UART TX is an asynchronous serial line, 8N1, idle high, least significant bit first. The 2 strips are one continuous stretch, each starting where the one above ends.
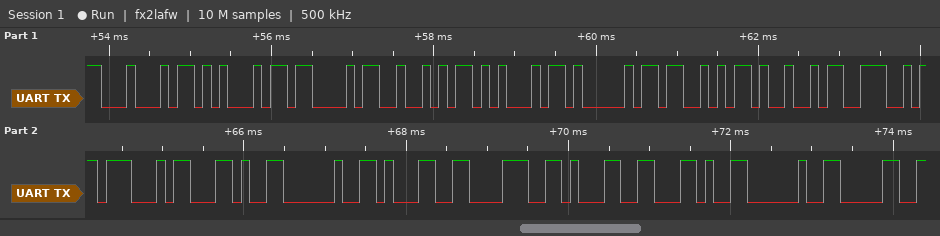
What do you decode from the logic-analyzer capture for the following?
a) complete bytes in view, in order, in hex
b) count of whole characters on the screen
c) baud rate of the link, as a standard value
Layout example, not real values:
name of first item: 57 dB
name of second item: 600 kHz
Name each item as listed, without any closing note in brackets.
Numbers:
complete bytes in view, in order, in hex: 0x44 0x45 0x43 0x52 0x45 0x41 0x53 0x49 0x4E 0x47 0x2C 0x20 0x31 0x38 0x31 0x2C 0x20 0x30
count of whole characters on the screen: 18
baud rate of the link, as a standard value: 9600 baud
